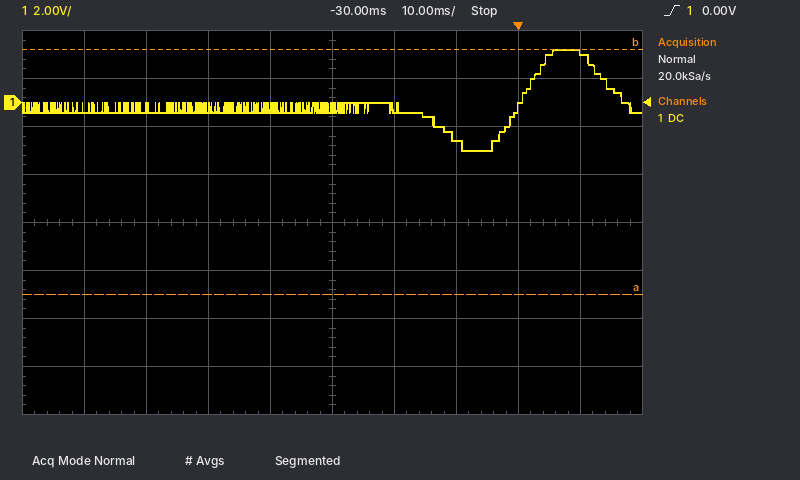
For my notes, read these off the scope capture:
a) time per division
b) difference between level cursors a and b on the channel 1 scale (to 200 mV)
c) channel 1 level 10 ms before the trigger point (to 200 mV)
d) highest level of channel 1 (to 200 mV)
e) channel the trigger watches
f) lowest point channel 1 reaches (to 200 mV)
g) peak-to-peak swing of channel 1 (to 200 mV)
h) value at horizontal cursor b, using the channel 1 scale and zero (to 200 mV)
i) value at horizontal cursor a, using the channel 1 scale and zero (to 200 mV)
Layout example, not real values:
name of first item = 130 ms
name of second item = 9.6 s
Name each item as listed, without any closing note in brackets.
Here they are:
time per division = 10 ms
difference between level cursors a and b on the channel 1 scale = 10.2 V
channel 1 level 10 ms before the trigger point = -1.6 V
highest level of channel 1 = 2.2 V
channel the trigger watches = channel 1
lowest point channel 1 reaches = -2.0 V
peak-to-peak swing of channel 1 = 4.2 V
value at horizontal cursor b, using the channel 1 scale and zero = 2.2 V
value at horizontal cursor a, using the channel 1 scale and zero = -8.0 V
